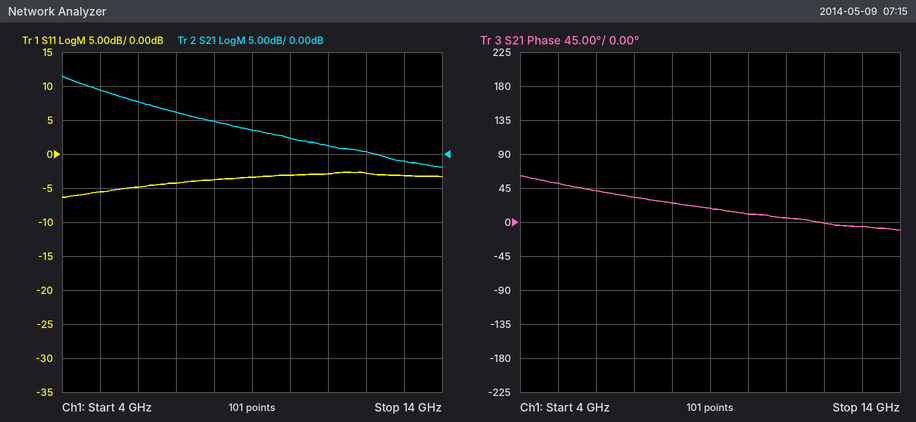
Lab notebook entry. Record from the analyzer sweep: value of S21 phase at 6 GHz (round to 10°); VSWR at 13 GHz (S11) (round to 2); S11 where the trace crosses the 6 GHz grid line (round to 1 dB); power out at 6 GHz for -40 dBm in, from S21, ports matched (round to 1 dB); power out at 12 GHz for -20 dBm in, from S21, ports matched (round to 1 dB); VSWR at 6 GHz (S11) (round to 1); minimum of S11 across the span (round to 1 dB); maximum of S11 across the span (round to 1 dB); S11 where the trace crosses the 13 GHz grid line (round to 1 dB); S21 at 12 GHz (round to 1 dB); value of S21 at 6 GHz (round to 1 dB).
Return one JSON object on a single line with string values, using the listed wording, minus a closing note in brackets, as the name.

{"value of S21 phase at 6 GHz": "40°", "VSWR at 13 GHz (S11)": "6", "S11 where the trace crosses the 6 GHz grid line": "-5 dB", "power out at 6 GHz for -40 dBm in, from S21, ports matched": "-32 dBm", "power out at 12 GHz for -20 dBm in, from S21, ports matched": "-20 dBm", "VSWR at 6 GHz (S11)": "4", "minimum of S11 across the span": "-6 dB", "maximum of S11 across the span": "-3 dB", "S11 where the trace crosses the 13 GHz grid line": "-3 dB", "S21 at 12 GHz": "0 dB", "value of S21 at 6 GHz": "8 dB"}
